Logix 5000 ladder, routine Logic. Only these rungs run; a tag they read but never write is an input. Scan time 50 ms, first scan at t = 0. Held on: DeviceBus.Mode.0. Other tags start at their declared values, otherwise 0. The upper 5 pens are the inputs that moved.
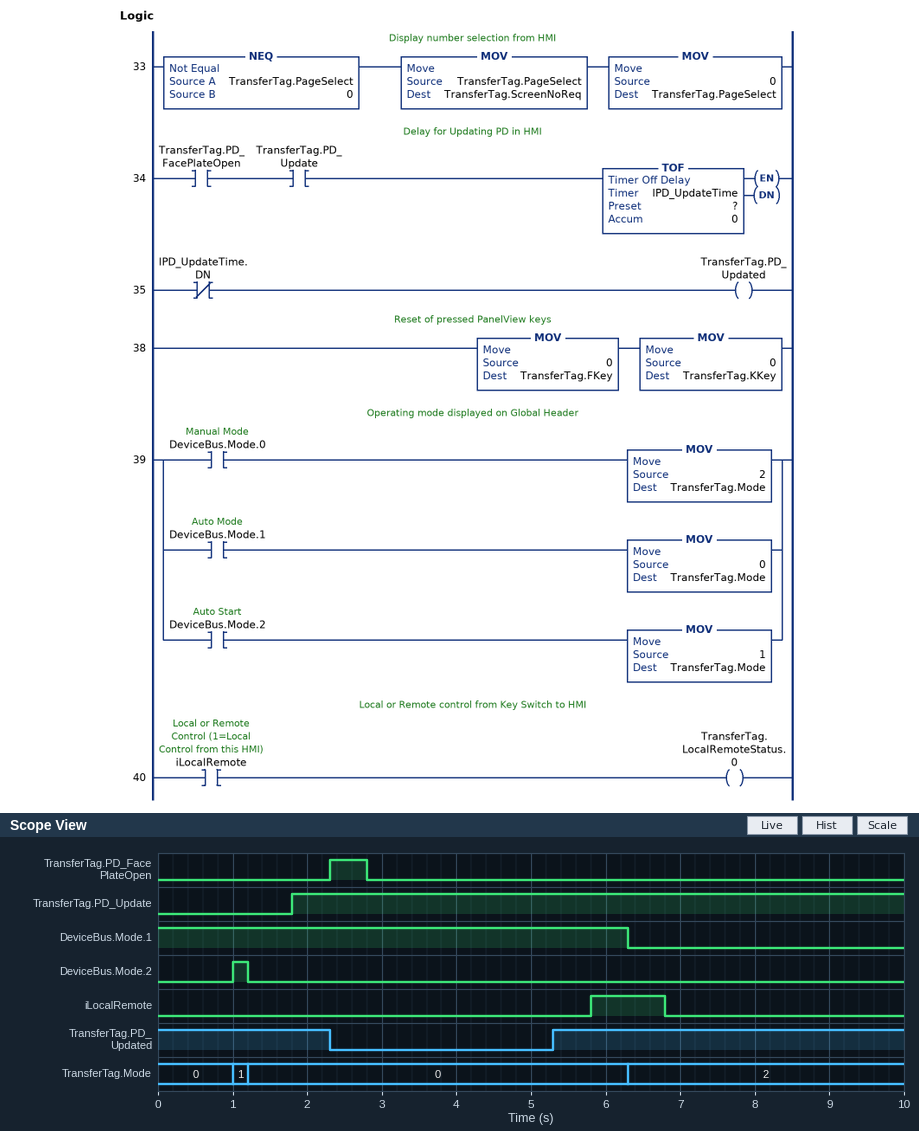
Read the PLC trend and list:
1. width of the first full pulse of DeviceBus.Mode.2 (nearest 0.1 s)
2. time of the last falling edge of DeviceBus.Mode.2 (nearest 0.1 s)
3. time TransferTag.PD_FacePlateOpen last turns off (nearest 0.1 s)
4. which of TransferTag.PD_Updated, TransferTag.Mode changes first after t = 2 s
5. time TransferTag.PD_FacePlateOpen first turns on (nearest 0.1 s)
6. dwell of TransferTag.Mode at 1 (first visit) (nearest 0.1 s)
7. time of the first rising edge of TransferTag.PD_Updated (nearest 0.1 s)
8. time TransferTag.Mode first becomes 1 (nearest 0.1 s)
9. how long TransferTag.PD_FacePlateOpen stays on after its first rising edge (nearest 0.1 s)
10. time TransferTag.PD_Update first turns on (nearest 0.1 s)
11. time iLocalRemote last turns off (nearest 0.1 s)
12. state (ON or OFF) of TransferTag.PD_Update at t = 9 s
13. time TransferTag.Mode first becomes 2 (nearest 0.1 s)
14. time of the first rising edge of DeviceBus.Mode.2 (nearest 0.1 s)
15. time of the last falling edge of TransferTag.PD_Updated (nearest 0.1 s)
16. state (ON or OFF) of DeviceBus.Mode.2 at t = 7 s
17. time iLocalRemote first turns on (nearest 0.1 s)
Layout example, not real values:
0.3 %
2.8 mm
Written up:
0.2 s
1.2 s
2.8 s
TransferTag.PD_Updated
2.3 s
0.2 s
5.3 s
1.0 s
0.5 s
1.8 s
6.8 s
ON
6.3 s
1.0 s
2.3 s
OFF
5.8 s
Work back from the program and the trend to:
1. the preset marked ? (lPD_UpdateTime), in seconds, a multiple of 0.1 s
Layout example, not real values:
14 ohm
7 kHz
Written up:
2.5 s
